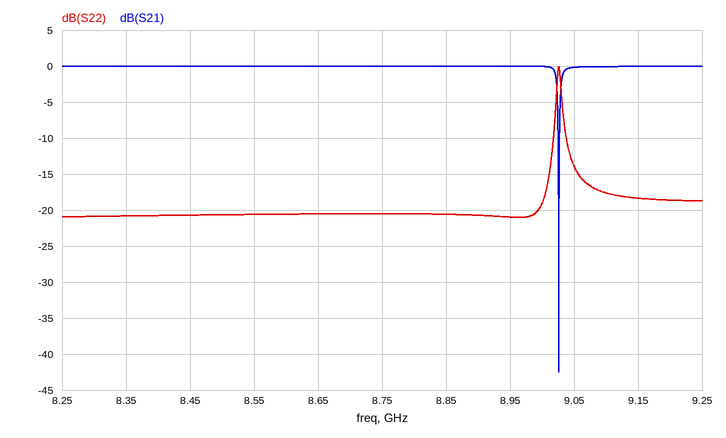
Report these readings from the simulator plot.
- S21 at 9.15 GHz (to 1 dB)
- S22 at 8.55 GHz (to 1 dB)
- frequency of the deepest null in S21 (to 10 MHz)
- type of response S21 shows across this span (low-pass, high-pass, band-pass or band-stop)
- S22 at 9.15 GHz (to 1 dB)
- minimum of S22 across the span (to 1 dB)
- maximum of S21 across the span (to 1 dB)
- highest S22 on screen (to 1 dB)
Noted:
0 dB
-21 dB
9.03 GHz
band-stop
-18 dB
-21 dB
0 dB
0 dB
